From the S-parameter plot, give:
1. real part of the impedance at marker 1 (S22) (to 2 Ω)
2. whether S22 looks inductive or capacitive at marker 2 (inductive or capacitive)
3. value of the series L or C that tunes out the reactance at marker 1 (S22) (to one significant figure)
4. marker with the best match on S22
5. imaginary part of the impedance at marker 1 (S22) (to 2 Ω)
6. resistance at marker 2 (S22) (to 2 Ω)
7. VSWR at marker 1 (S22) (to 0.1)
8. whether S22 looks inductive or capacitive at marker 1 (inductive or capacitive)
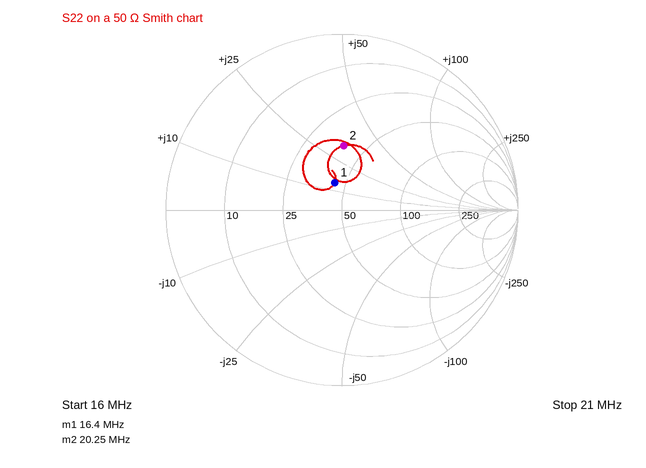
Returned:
44 Ω
inductive
700 pF
marker 1
+14 Ω
38 Ω
1.4
inductive
